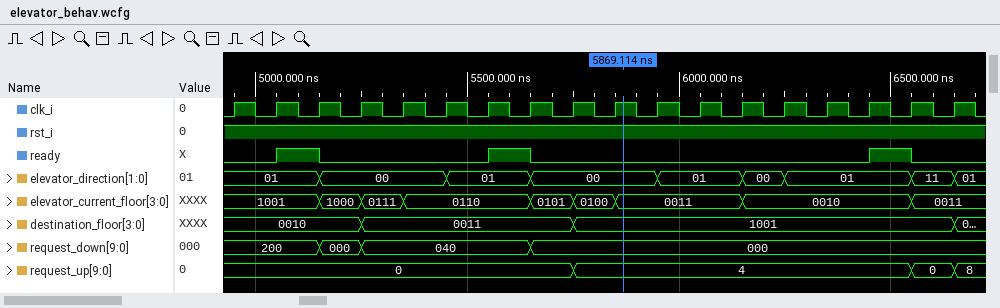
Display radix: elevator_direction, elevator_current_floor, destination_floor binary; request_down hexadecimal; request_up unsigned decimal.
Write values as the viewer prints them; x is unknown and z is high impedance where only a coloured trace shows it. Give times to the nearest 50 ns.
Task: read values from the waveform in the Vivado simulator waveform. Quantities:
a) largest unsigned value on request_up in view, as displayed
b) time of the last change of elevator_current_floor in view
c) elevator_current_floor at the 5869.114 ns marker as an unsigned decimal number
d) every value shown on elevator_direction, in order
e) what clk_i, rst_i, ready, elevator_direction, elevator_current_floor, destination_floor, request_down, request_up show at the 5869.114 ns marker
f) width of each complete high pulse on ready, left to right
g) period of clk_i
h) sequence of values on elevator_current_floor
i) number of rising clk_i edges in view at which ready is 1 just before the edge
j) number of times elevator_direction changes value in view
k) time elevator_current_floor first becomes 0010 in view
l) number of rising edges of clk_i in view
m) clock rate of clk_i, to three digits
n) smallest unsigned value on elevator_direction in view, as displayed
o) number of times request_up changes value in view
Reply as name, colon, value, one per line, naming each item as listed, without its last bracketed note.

largest unsigned value on request_up in view, as displayed: 8
time of the last change of elevator_current_floor in view: 6550 ns
elevator_current_floor at the 5869.114 ns marker as an unsigned decimal number: 3
every value shown on elevator_direction, in order: 01, 00, 01, 00, 01, 00, 01, 11, 01
what clk_i, rst_i, ready, elevator_direction, elevator_current_floor, destination_floor, request_down, request_up show at the 5869.114 ns marker: clk_i=1, rst_i=1, ready=0, elevator_direction=00, elevator_current_floor=0011, destination_floor=1001, request_down=000, request_up=4
width of each complete high pulse on ready, left to right: 100 ns, 100 ns, 100 ns
period of clk_i: 100 ns
sequence of values on elevator_current_floor: 1001, 1000, 0111, 0110, 0101, 0100, 0011, 0010, 0011
number of rising clk_i edges in view at which ready is 1 just before the edge: 3
number of times elevator_direction changes value in view: 8
time elevator_current_floor first becomes 0010 in view: 6150 ns
number of rising edges of clk_i in view: 18
clock rate of clk_i, to three digits: 10.0 MHz
smallest unsigned value on elevator_direction in view, as displayed: 00
number of times request_up changes value in view: 3
